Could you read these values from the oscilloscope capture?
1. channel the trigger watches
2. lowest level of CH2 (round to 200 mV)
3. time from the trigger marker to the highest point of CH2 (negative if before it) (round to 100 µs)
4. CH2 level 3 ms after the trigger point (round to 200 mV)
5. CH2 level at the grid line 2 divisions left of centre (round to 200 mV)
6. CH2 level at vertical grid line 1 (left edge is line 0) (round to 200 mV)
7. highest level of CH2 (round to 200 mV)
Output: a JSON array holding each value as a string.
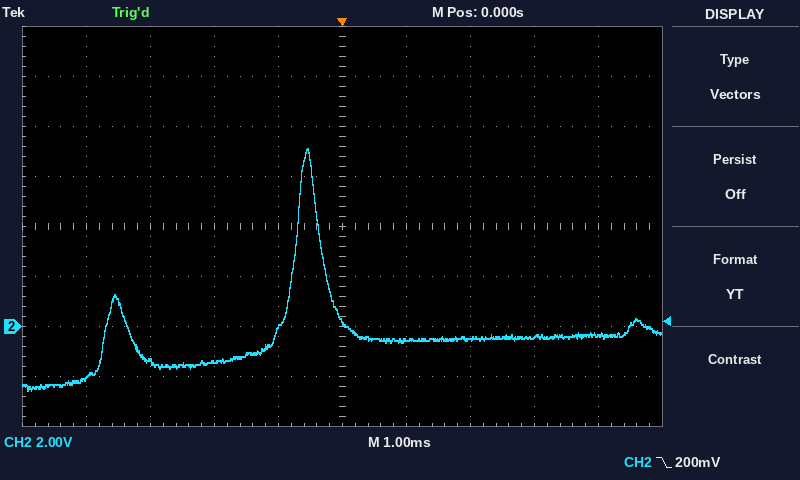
["CH2", "-2.6 V", "-500 µs", "-400 mV", "-1.4 V", "-2.0 V", "7.2 V"]
